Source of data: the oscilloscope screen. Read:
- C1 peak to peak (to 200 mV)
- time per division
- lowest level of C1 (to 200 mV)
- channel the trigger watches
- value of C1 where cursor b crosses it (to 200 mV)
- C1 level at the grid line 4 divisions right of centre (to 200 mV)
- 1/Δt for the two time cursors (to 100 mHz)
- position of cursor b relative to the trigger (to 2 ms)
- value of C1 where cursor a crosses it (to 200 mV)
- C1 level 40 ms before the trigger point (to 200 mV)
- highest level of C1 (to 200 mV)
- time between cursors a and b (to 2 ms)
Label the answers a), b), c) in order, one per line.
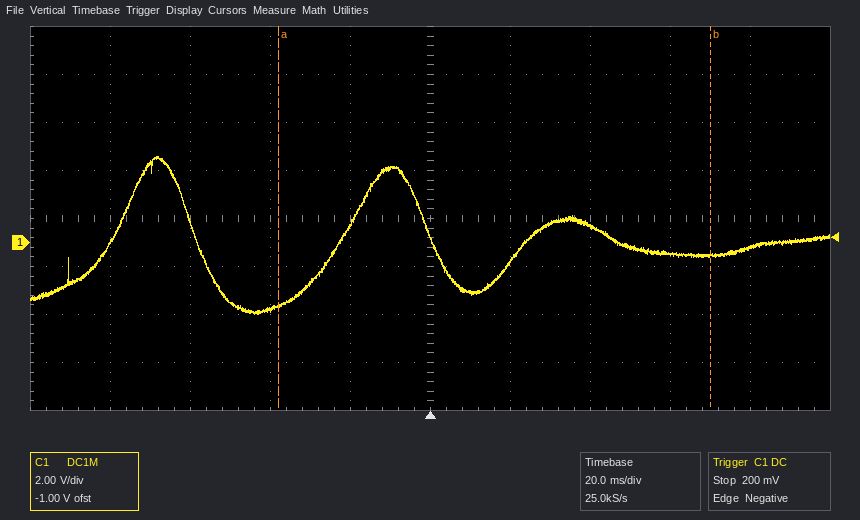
a) 6.6 V
b) 20 ms
c) -3.0 V
d) C1
e) -600 mV
f) -200 mV
g) 9.3 Hz
h) +70 ms
i) -2.6 V
j) -2.8 V
k) 3.6 V
l) 108 ms
